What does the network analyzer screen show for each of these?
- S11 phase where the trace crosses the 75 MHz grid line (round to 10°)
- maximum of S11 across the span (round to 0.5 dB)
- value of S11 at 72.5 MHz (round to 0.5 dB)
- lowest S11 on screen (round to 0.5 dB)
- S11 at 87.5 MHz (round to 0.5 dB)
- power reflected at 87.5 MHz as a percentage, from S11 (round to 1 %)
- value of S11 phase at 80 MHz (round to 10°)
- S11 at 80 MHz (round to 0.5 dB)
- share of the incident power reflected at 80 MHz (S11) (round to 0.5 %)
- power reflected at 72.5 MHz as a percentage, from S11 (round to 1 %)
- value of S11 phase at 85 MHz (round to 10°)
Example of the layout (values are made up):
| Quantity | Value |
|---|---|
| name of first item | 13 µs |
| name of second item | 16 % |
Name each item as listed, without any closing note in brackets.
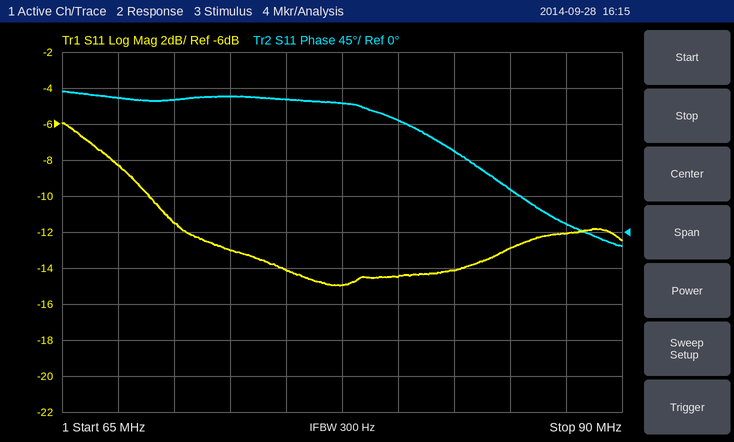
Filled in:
| Quantity | Value |
|---|---|
| S11 phase where the trace crosses the 75 MHz grid line | 170° |
| maximum of S11 across the span | -6.0 dB |
| value of S11 at 72.5 MHz | -13.0 dB |
| lowest S11 on screen | -15.0 dB |
| S11 at 87.5 MHz | -12.0 dB |
| power reflected at 87.5 MHz as a percentage, from S11 | 6 % |
| value of S11 phase at 80 MHz | 140° |
| S11 at 80 MHz | -14.5 dB |
| share of the incident power reflected at 80 MHz (S11) | 3.5 % |
| power reflected at 72.5 MHz as a percentage, from S11 | 5 % |
| value of S11 phase at 85 MHz | 50° |
